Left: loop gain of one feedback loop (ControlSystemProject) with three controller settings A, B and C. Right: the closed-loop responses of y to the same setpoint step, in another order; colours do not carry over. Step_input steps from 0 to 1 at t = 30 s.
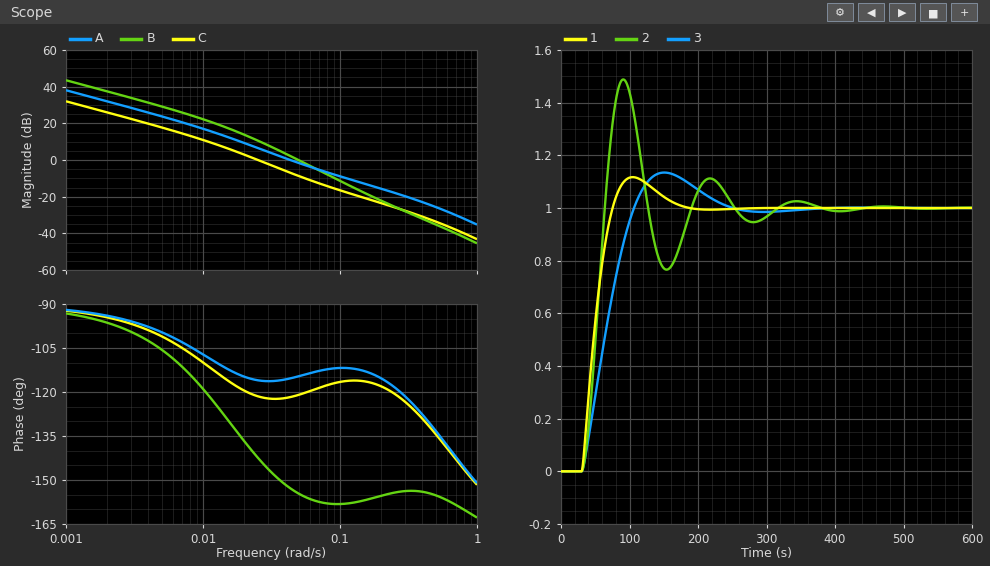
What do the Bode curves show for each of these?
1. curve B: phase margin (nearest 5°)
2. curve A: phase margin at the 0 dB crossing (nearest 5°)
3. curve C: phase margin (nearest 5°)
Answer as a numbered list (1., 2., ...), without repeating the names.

1. 25°
2. 65°
3. 60°
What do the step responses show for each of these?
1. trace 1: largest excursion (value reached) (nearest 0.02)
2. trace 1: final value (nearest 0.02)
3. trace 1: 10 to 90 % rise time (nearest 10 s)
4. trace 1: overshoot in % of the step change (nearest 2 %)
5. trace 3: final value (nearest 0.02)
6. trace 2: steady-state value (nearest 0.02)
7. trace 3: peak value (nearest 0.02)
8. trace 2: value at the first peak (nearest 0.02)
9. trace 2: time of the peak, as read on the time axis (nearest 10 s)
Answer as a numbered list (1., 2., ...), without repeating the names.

1. 1.12
2. 1.00
3. 30 s
4. 12 %
5. 1.00
6. 1.00
7. 1.14
8. 1.48
9. 90 s
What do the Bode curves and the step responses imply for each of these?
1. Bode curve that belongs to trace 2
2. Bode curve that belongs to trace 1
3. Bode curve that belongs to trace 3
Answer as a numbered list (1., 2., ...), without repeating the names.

1. B
2. A
3. C
